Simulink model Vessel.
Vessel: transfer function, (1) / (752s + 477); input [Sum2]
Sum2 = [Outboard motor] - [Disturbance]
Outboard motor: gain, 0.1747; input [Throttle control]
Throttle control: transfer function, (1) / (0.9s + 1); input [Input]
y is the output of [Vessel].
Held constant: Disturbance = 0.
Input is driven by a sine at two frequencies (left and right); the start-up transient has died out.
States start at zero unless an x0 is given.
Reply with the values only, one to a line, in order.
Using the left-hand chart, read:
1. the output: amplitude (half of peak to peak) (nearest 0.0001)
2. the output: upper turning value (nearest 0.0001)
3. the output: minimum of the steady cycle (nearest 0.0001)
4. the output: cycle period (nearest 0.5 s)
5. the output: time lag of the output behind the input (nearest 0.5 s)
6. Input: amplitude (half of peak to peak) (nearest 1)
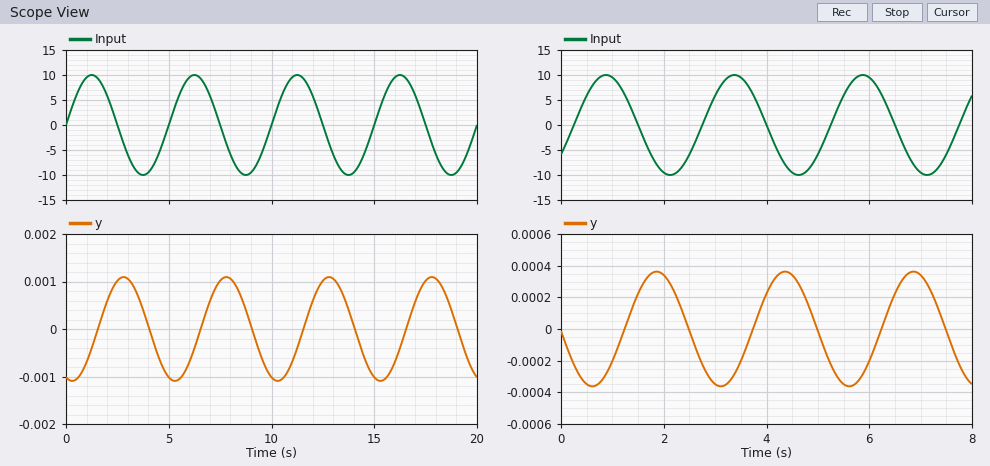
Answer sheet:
0.0011
0.0011
-0.0011
5.0 s
1.5 s
10
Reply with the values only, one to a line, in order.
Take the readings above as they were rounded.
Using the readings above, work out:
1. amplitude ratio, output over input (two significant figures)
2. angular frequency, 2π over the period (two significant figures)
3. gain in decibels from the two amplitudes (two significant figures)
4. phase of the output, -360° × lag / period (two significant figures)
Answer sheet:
0.00011
1.3 rad/s
-79 dB
-110°
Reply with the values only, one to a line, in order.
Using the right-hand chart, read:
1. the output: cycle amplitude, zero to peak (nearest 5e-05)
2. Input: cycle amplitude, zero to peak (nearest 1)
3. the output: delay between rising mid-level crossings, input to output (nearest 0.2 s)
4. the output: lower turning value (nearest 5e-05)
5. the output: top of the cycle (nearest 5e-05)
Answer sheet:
0.00035
10
1.0 s
-0.00035
0.00035
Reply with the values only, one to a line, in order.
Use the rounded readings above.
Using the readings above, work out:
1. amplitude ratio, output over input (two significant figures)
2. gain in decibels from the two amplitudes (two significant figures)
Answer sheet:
0.000035
-89 dB
